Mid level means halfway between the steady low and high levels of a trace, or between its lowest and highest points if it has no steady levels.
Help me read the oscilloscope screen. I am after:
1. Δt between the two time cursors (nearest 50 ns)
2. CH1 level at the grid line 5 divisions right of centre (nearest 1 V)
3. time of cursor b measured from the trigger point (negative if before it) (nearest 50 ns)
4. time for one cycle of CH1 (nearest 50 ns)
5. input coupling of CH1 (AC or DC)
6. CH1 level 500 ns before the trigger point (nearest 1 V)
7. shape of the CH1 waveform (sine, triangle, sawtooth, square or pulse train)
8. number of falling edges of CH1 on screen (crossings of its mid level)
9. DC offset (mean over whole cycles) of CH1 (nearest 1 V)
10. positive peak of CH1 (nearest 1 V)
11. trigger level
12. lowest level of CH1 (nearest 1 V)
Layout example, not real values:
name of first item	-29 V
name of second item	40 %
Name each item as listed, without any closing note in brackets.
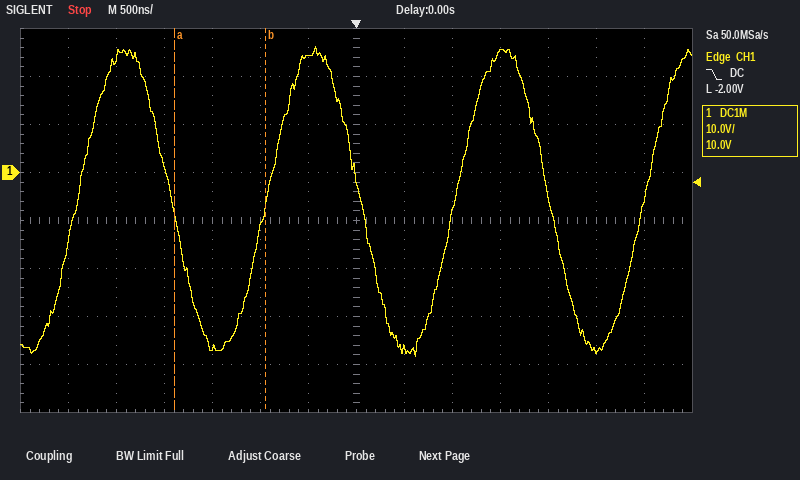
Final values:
Δt between the two time cursors	950 ns
CH1 level at the grid line 5 divisions right of centre	-37 V
time of cursor b measured from the trigger point (negative if before it)	-950 ns
time for one cycle of CH1	1.95 µs
input coupling of CH1	DC
CH1 level 500 ns before the trigger point	24 V
shape of the CH1 waveform	sine
number of falling edges of CH1 on screen	3
DC offset (mean over whole cycles) of CH1	-6 V
positive peak of CH1	26 V
trigger level	-2.00 V
lowest level of CH1	-38 V
